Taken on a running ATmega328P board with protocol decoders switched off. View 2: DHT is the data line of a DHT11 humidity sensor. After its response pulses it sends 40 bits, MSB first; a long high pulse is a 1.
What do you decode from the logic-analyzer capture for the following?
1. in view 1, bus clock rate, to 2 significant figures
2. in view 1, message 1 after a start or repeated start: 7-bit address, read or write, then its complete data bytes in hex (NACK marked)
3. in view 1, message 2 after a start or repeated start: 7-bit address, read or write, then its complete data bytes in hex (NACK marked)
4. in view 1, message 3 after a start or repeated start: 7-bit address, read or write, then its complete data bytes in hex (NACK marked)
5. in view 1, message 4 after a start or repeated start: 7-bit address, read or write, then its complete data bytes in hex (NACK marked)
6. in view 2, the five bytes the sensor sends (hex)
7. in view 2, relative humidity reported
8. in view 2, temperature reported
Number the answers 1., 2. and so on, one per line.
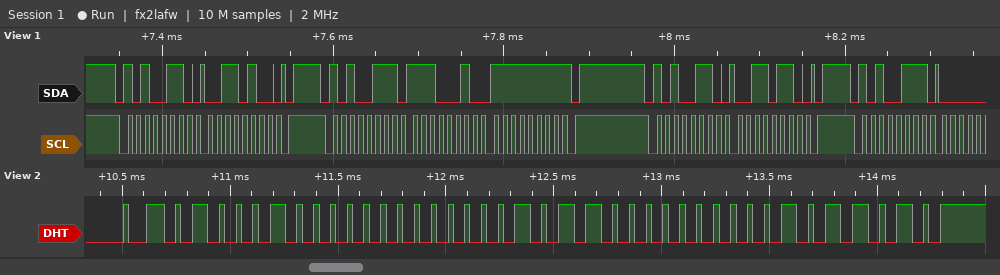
1. 100 kHz
2. 0x53 write: 34
3. 0x53 read: E2 FF NACK
4. 0x53 write: 36
5. 0x53 read
6. 44 00 16 00 5A
7. 68 %
8. 22.0 °C
